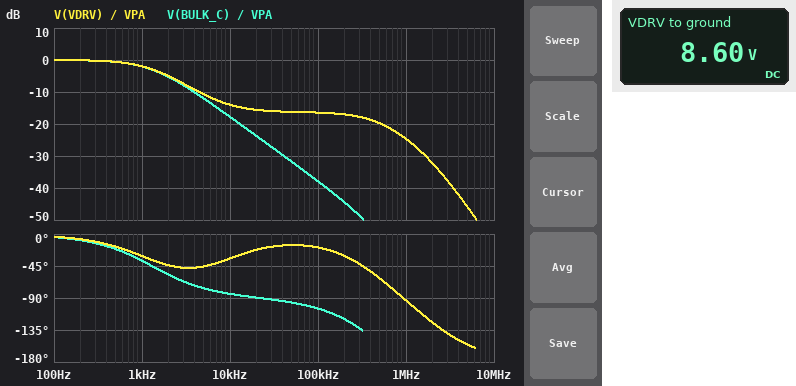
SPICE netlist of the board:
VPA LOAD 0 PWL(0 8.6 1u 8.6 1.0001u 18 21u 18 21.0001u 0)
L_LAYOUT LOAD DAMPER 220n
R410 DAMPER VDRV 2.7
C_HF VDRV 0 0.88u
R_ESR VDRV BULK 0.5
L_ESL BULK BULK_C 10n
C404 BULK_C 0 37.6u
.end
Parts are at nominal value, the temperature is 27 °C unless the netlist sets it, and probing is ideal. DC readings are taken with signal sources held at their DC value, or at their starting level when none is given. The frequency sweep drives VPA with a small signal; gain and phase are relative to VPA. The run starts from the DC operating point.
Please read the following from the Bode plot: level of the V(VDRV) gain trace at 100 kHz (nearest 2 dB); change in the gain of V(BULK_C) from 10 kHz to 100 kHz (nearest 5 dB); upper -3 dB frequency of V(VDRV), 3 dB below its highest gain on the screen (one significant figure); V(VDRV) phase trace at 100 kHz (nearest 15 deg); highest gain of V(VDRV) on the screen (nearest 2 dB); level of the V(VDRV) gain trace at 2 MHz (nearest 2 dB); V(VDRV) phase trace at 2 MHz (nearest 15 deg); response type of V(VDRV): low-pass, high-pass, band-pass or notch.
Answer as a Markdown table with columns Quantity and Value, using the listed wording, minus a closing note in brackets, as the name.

| Quantity | Value |
|---|---|
| level of the V(VDRV) gain trace at 100 kHz | -16 dB |
| change in the gain of V(BULK_C) from 10 kHz to 100 kHz | -20 dB |
| upper -3 dB frequency of V(VDRV), 3 dB below its highest gain on the screen | 1 kHz |
| V(VDRV) phase trace at 100 kHz | -15 deg |
| highest gain of V(VDRV) on the screen | 0 dB |
| level of the V(VDRV) gain trace at 2 MHz | -32 dB |
| V(VDRV) phase trace at 2 MHz | -120 deg |
| response type of V(VDRV): low-pass, high-pass, band-pass or notch | low-pass |
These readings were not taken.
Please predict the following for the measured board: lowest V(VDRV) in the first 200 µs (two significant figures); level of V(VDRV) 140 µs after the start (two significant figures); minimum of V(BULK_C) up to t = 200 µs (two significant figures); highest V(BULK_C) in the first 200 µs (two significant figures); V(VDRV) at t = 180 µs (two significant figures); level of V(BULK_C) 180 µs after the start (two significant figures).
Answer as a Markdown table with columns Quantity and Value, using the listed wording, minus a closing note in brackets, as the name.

| Quantity | Value |
|---|---|
| lowest V(VDRV) in the first 200 µs | 2.0 V |
| level of V(VDRV) 140 µs after the start | 3.2 V |
| minimum of V(BULK_C) up to t = 200 µs | 2.3 V |
| highest V(BULK_C) in the first 200 µs | 10 V |
| V(VDRV) at t = 180 µs | 2.3 V |
| level of V(BULK_C) 180 µs after the start | 2.7 V |
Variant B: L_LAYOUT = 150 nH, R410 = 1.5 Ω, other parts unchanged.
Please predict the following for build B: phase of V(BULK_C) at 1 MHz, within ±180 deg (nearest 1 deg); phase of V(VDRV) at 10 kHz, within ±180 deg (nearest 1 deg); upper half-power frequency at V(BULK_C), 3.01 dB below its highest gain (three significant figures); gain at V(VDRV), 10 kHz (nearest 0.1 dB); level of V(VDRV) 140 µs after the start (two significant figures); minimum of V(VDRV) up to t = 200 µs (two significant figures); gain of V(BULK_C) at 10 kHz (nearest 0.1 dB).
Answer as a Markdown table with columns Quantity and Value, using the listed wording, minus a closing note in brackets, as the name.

| Quantity | Value |
|---|---|
| phase of V(BULK_C) at 1 MHz, within ±180 deg | 167 deg |
| phase of V(VDRV) at 10 kHz, within ±180 deg | -30 deg |
| upper half-power frequency at V(BULK_C), 3.01 dB below its highest gain | 2.09 kHz |
| gain at V(VDRV), 10 kHz | -10.0 dB |
| level of V(VDRV) 140 µs after the start | 1.7 V |
| minimum of V(VDRV) up to t = 200 µs | 780 mV |
| gain of V(BULK_C) at 10 kHz | -13.8 dB |
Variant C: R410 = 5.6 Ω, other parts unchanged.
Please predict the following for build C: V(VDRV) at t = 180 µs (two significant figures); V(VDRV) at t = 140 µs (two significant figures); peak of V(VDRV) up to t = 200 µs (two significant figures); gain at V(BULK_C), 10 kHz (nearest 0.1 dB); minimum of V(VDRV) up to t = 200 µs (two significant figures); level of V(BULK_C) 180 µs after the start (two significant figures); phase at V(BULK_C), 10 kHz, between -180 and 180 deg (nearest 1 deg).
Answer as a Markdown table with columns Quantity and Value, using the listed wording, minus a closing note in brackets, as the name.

| Quantity | Value |
|---|---|
| V(VDRV) at t = 180 µs | 4.4 V |
| V(VDRV) at t = 140 µs | 5.2 V |
| peak of V(VDRV) up to t = 200 µs | 10 V |
| gain at V(BULK_C), 10 kHz | -23.4 dB |
| minimum of V(VDRV) up to t = 200 µs | 4.0 V |
| level of V(BULK_C) 180 µs after the start | 4.8 V |
| phase at V(BULK_C), 10 kHz, between -180 and 180 deg | -88 deg |
